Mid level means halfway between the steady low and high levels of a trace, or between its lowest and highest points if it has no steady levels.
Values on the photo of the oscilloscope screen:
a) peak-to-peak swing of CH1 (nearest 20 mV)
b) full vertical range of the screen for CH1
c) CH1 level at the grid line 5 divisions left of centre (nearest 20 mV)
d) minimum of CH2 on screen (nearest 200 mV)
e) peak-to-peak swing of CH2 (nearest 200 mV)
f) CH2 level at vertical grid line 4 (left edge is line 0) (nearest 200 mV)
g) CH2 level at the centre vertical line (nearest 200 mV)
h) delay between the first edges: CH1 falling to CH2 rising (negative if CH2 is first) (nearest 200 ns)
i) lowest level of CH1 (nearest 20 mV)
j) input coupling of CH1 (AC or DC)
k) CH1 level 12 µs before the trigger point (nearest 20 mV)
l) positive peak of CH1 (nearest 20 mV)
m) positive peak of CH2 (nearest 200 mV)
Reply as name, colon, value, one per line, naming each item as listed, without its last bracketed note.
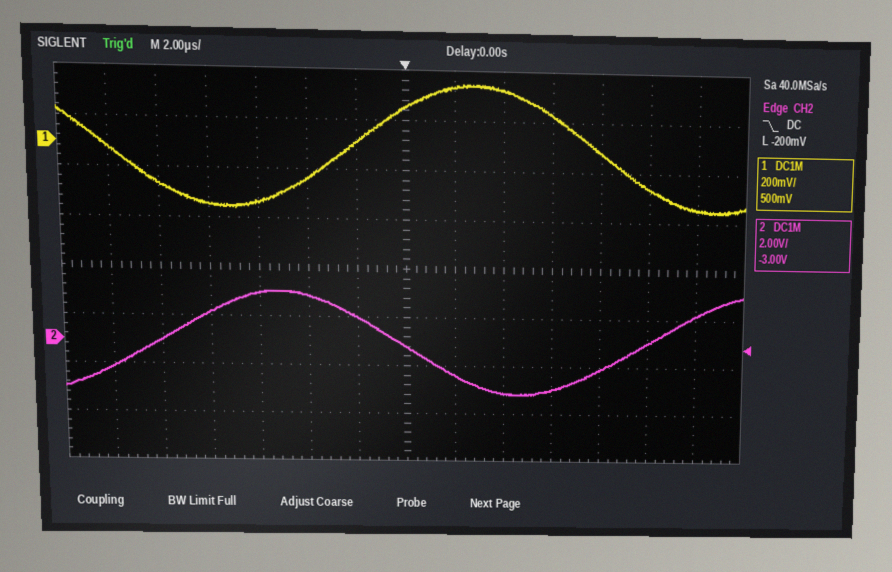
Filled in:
peak-to-peak swing of CH1: 500 mV
full vertical range of the screen for CH1: 1.6 V
CH1 level at the grid line 5 divisions left of centre: -160 mV
minimum of CH2 on screen: -2.2 V
peak-to-peak swing of CH2: 4.2 V
CH2 level at vertical grid line 4 (left edge is line 0): 2.0 V
CH2 level at the centre vertical line: -200 mV
delay between the first edges: CH1 falling to CH2 rising (negative if CH2 is first): +2.0 µs
lowest level of CH1: -260 mV
input coupling of CH1: DC
CH1 level 12 µs before the trigger point: -20 mV
positive peak of CH1: 240 mV
positive peak of CH2: 2.0 V
